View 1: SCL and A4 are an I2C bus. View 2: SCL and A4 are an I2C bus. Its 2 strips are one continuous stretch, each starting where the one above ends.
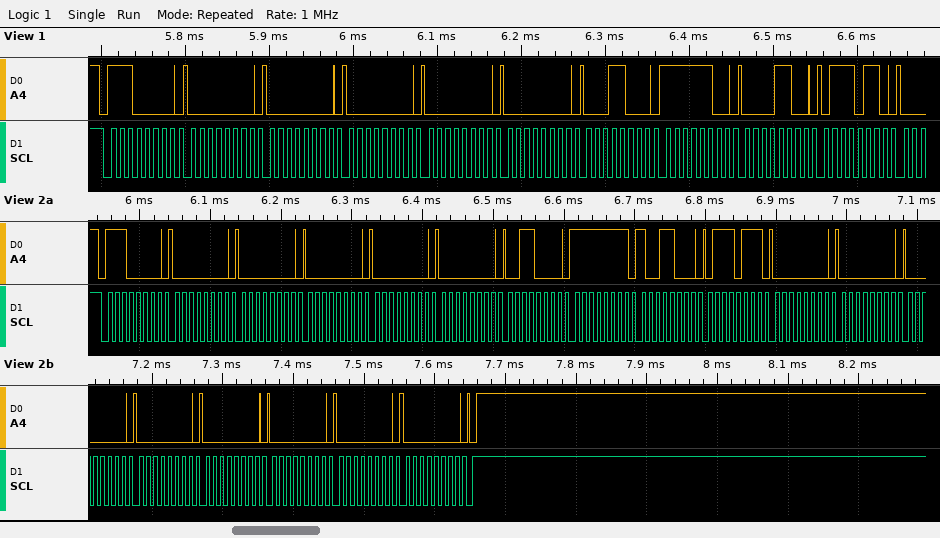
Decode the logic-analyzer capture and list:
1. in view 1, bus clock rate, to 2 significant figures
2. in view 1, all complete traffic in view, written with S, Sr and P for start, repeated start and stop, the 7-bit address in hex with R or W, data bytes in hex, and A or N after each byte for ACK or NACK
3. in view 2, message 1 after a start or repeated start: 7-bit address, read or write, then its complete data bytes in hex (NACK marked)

100 kHz
S 70W A 00 A 00 A 00 A 00 A 00 A 18 A FC A 0C A 76 A
0x70 write: 00 00 00 00 00 30 FF 98 77 00 00 00 00 00 00 00 00
